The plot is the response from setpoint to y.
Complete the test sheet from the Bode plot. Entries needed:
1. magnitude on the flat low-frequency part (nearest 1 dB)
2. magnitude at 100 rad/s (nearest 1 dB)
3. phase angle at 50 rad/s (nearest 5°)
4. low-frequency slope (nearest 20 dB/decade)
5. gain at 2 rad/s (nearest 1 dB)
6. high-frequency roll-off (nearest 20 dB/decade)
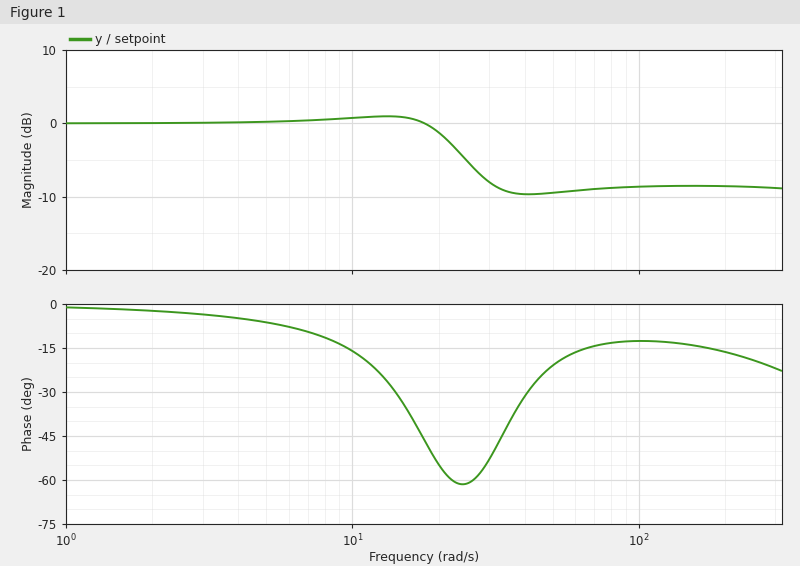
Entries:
0 dB
-9 dB
-20°
0 dB/decade
0 dB
0 dB/decade
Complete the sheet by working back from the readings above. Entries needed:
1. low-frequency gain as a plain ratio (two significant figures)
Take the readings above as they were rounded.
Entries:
1.0
